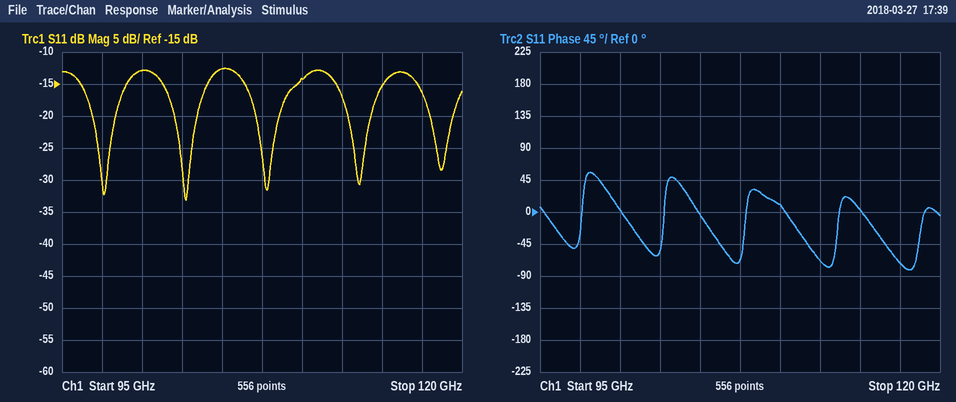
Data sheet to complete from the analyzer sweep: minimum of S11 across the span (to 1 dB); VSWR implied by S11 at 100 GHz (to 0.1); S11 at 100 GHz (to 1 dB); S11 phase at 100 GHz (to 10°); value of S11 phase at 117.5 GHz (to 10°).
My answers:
-33 dB
1.6
-13 dB
0°
-70°
